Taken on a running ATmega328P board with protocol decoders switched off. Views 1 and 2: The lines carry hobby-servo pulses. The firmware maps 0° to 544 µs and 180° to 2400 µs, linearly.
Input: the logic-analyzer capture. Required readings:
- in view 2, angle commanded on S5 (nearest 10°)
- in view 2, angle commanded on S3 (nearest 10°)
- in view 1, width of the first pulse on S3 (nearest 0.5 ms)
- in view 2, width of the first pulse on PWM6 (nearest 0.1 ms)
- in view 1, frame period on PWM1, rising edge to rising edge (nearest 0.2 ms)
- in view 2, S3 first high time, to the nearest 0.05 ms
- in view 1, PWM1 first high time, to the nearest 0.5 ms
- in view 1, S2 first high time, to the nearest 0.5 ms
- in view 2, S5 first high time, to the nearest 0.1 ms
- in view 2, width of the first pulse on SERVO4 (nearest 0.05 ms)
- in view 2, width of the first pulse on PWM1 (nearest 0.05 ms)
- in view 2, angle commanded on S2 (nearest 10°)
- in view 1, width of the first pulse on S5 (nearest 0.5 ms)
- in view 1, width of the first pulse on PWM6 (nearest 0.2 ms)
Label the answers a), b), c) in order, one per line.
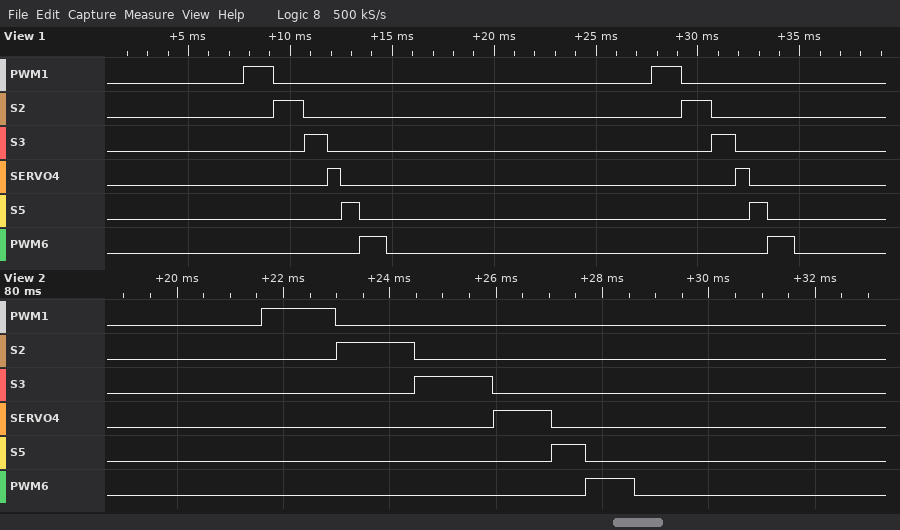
a) 10°
b) 90°
c) 1.0 ms
d) 0.9 ms
e) 20.0 ms
f) 1.45 ms
g) 1.5 ms
h) 1.5 ms
i) 0.6 ms
j) 1.10 ms
k) 1.40 ms
l) 90°
m) 1.0 ms
n) 1.4 ms
